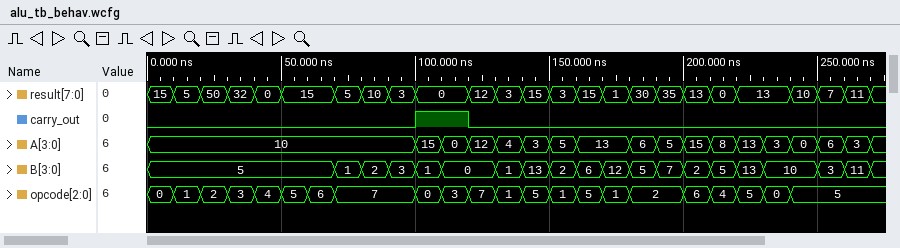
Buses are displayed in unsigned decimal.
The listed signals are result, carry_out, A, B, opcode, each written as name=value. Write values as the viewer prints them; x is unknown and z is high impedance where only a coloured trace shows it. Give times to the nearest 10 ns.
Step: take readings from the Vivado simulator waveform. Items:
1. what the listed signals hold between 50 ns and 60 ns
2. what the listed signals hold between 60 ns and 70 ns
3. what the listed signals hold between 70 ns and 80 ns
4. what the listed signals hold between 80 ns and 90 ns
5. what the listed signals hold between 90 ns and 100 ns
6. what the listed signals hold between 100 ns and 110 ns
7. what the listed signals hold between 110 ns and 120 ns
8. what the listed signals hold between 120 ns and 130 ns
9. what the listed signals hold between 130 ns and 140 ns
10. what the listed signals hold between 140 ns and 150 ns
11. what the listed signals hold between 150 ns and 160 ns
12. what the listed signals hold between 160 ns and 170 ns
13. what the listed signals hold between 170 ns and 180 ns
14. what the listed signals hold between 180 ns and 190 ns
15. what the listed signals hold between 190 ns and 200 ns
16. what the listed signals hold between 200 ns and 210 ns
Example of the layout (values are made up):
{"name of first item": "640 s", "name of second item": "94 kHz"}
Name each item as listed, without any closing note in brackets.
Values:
{"what the listed signals hold between 50 ns and 60 ns": "result=15, carry_out=0, A=10, B=5, opcode=5", "what the listed signals hold between 60 ns and 70 ns": "result=15, carry_out=0, A=10, B=5, opcode=6", "what the listed signals hold between 70 ns and 80 ns": "result=5, carry_out=0, A=10, B=1, opcode=7", "what the listed signals hold between 80 ns and 90 ns": "result=10, carry_out=0, A=10, B=2, opcode=7", "what the listed signals hold between 90 ns and 100 ns": "result=3, carry_out=0, A=10, B=3, opcode=7", "what the listed signals hold between 100 ns and 110 ns": "result=0, carry_out=1, A=15, B=1, opcode=0", "what the listed signals hold between 110 ns and 120 ns": "result=0, carry_out=1, A=0, B=0, opcode=3", "what the listed signals hold between 120 ns and 130 ns": "result=12, carry_out=0, A=12, B=0, opcode=7", "what the listed signals hold between 130 ns and 140 ns": "result=3, carry_out=0, A=4, B=1, opcode=1", "what the listed signals hold between 140 ns and 150 ns": "result=15, carry_out=0, A=3, B=13, opcode=5", "what the listed signals hold between 150 ns and 160 ns": "result=3, carry_out=0, A=5, B=2, opcode=1", "what the listed signals hold between 160 ns and 170 ns": "result=15, carry_out=0, A=13, B=6, opcode=5", "what the listed signals hold between 170 ns and 180 ns": "result=1, carry_out=0, A=13, B=12, opcode=1", "what the listed signals hold between 180 ns and 190 ns": "result=30, carry_out=0, A=6, B=5, opcode=2", "what the listed signals hold between 190 ns and 200 ns": "result=35, carry_out=0, A=5, B=7, opcode=2", "what the listed signals hold between 200 ns and 210 ns": "result=13, carry_out=0, A=15, B=2, opcode=6"}
